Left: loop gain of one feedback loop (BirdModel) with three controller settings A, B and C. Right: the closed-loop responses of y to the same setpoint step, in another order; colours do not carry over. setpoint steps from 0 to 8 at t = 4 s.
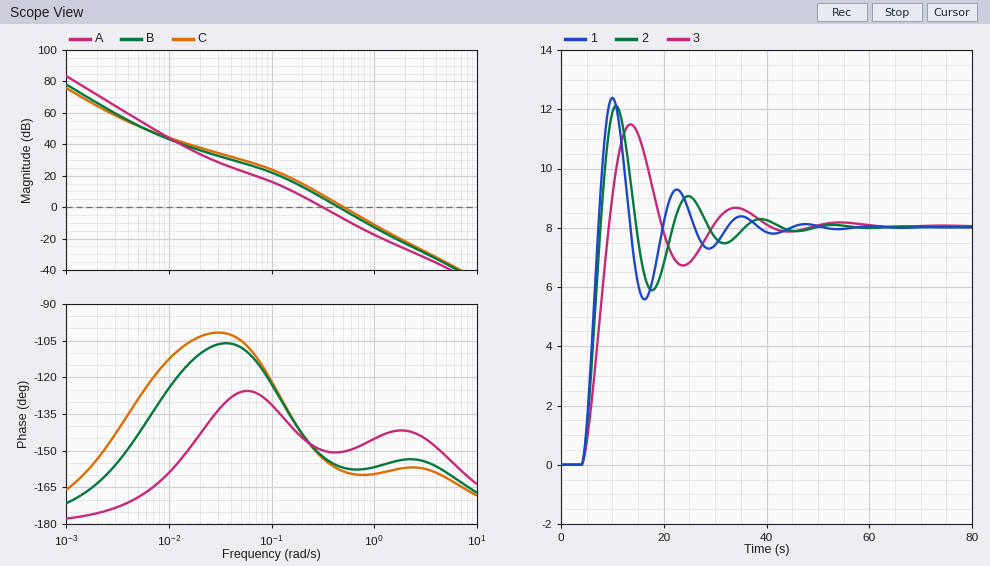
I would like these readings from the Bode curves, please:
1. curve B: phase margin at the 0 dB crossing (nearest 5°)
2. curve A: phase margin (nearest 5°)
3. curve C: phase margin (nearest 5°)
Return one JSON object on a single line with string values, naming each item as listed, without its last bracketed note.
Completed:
{"curve B: phase margin at the 0 dB crossing": "25°", "curve A: phase margin": "30°", "curve C: phase margin": "20°"}
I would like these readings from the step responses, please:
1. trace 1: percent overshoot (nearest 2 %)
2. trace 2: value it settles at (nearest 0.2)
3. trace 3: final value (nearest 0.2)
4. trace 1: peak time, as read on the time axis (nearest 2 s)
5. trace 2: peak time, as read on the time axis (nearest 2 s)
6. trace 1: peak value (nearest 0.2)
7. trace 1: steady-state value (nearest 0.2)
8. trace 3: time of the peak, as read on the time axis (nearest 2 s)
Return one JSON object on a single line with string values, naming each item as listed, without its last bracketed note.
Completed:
{"trace 1: percent overshoot": "54 %", "trace 2: value it settles at": "8.0", "trace 3: final value": "8.0", "trace 1: peak time, as read on the time axis": "10 s", "trace 2: peak time, as read on the time axis": "10 s", "trace 1: peak value": "12.4", "trace 1: steady-state value": "8.0", "trace 3: time of the peak, as read on the time axis": "14 s"}
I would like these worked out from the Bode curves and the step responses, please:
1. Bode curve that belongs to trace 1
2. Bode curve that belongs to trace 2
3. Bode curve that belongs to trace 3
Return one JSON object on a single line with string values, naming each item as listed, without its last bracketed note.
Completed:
{"Bode curve that belongs to trace 1": "C", "Bode curve that belongs to trace 2": "B", "Bode curve that belongs to trace 3": "A"}
